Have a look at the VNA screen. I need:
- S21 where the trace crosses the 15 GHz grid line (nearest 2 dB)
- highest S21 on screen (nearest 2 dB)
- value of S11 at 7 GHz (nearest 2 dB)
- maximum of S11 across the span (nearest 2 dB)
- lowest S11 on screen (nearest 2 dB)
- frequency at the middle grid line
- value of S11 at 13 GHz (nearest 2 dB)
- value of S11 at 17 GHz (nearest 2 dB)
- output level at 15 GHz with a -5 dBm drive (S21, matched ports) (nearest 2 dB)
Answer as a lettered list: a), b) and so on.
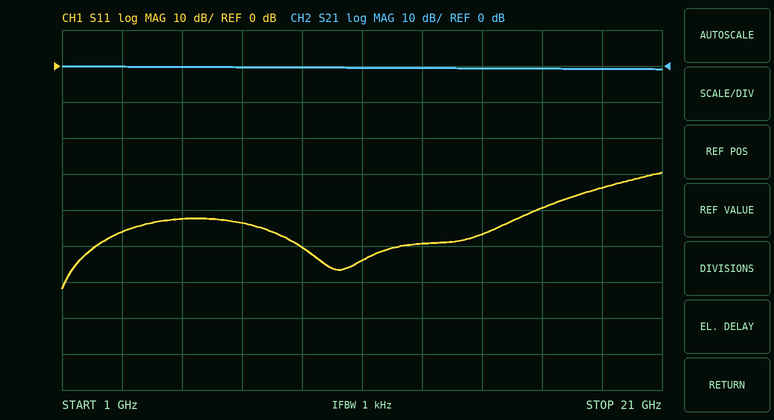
a) 0 dB
b) 0 dB
c) -44 dB
d) -30 dB
e) -62 dB
f) 11 GHz
g) -50 dB
h) -40 dB
i) -6 dBm
